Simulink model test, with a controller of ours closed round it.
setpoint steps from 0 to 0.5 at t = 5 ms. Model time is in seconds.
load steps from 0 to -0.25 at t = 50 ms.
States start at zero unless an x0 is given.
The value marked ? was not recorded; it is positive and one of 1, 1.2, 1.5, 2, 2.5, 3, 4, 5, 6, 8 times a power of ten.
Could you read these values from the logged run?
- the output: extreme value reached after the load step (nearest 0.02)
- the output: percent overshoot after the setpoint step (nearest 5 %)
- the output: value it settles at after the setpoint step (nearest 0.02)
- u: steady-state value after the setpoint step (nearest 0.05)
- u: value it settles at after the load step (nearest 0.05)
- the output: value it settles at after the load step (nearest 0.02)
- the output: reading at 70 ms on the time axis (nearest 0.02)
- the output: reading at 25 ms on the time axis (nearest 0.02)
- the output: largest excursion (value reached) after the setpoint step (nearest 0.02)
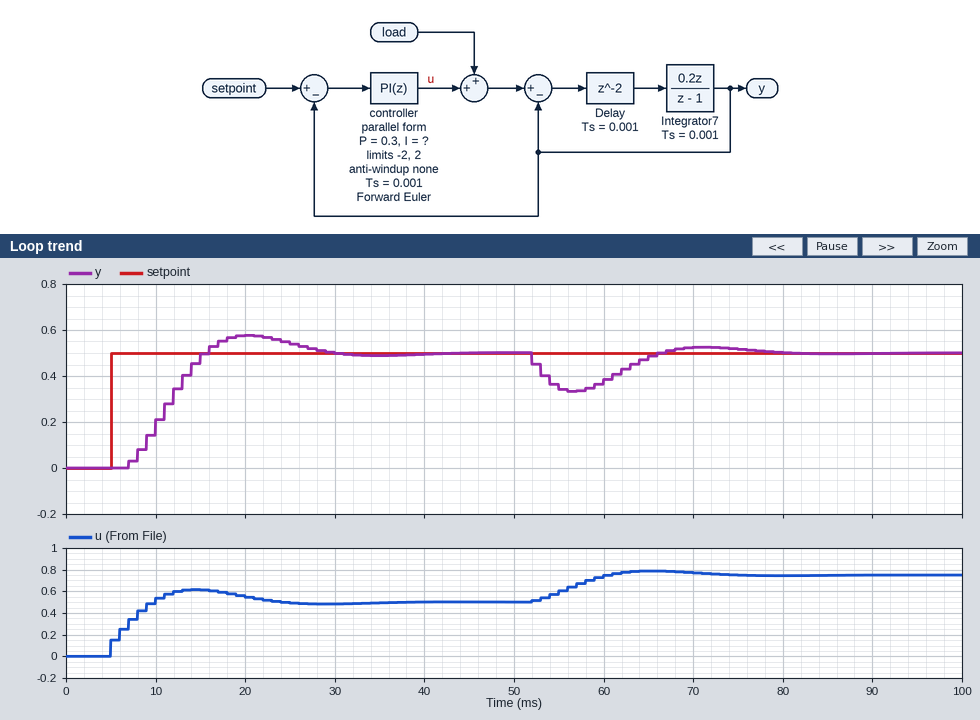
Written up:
0.34
15 %
0.50
0.50
0.75
0.50
0.52
0.54
0.58
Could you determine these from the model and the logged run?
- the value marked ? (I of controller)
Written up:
200
